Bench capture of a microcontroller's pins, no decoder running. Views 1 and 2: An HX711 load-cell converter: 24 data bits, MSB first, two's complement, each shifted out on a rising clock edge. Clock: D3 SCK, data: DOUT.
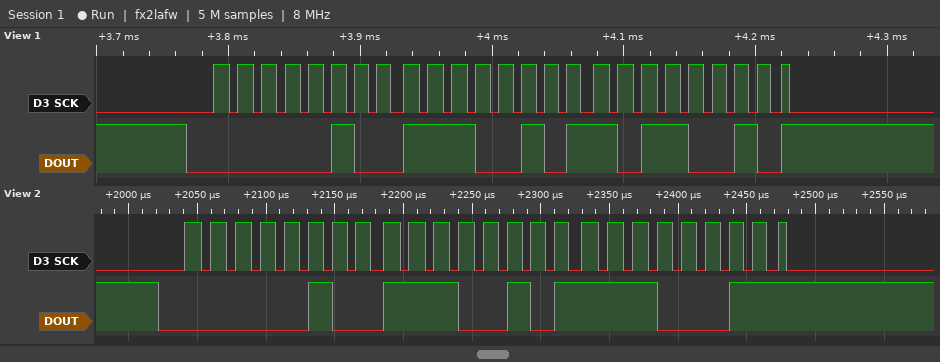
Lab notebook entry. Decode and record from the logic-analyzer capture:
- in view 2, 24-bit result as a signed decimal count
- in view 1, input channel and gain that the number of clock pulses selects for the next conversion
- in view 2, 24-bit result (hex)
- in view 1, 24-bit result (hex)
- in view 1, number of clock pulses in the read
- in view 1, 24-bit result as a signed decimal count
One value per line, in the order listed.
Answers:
320995
channel A, gain 128
0x04E5E3
0x04E5B2
25
320946
